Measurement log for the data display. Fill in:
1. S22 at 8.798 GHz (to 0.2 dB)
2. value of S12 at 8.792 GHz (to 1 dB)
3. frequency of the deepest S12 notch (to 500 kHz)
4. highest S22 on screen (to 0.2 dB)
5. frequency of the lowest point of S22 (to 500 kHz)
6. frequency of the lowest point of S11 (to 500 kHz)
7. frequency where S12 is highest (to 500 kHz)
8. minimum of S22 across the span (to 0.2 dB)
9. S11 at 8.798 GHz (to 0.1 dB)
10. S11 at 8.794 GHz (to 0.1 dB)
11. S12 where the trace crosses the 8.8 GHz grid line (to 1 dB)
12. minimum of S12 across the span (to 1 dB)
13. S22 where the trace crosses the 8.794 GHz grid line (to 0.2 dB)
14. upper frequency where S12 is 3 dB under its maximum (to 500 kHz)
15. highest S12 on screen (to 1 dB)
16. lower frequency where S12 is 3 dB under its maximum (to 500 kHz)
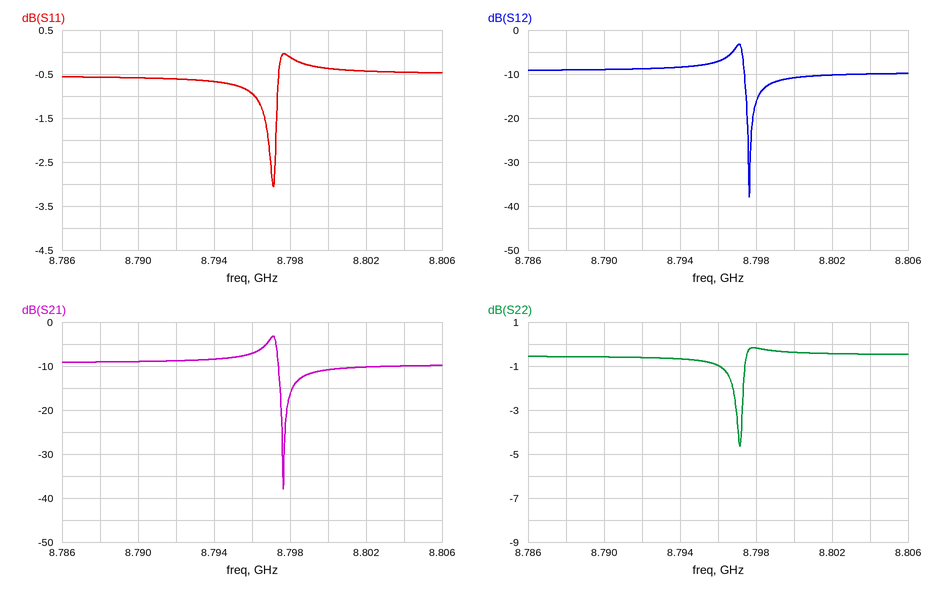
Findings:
-0.2 dB
-9 dB
8.7975 GHz
-0.2 dB
8.7970 GHz
8.7970 GHz
8.7970 GHz
-4.6 dB
-0.1 dB
-0.7 dB
-11 dB
-38 dB
-0.6 dB
8.7975 GHz
-3 dB
8.7965 GHz
